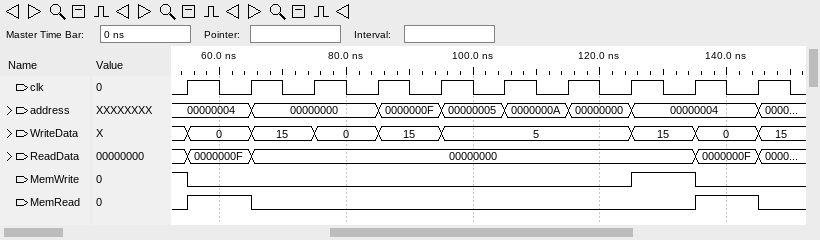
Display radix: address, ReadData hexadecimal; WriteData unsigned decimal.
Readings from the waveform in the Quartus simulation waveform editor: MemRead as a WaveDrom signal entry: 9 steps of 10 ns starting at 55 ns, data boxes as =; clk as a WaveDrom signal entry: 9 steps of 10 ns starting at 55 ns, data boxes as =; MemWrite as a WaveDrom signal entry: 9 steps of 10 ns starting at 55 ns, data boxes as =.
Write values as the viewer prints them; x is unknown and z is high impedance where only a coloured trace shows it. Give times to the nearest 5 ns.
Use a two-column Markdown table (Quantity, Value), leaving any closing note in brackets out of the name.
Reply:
| Quantity | Value |
|---|---|
| MemRead as a WaveDrom signal entry: 9 steps of 10 ns starting at 55 ns, data boxes as = | {name: 'MemRead', wave: '10......1'} |
| clk as a WaveDrom signal entry: 9 steps of 10 ns starting at 55 ns, data boxes as = | {name: 'clk', wave: 'p........'} |
| MemWrite as a WaveDrom signal entry: 9 steps of 10 ns starting at 55 ns, data boxes as = | {name: 'MemWrite', wave: '0......10'} |
